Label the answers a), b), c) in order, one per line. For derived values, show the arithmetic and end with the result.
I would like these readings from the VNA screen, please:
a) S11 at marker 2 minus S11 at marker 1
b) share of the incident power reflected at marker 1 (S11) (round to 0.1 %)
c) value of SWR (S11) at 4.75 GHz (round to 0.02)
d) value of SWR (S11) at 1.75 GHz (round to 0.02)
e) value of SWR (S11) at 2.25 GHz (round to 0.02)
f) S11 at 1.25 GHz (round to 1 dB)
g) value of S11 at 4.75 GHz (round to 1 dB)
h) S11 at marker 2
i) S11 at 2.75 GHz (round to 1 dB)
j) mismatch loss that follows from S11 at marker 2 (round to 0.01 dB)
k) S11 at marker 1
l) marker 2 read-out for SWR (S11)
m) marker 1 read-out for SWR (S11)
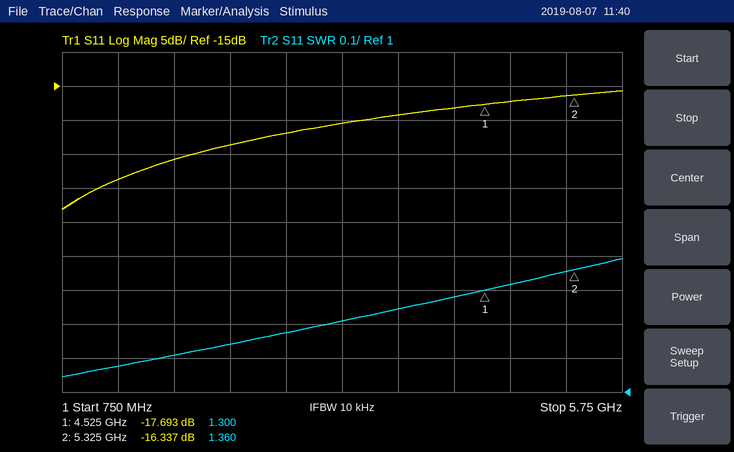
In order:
a) -16.337 − (-17.693) = 1.356 dB
b) 10^(-17.693/10) ≈ 1.7 %
c) 1.32
d) 1.10
e) 1.14
f) -29 dB
g) -17 dB
h) -16.337 dB
i) -22 dB
j) −10 log10(1 − 10^(-16.337/10)) ≈ 0.10 dB
k) -17.693 dB
l) 1.360
m) 1.300
